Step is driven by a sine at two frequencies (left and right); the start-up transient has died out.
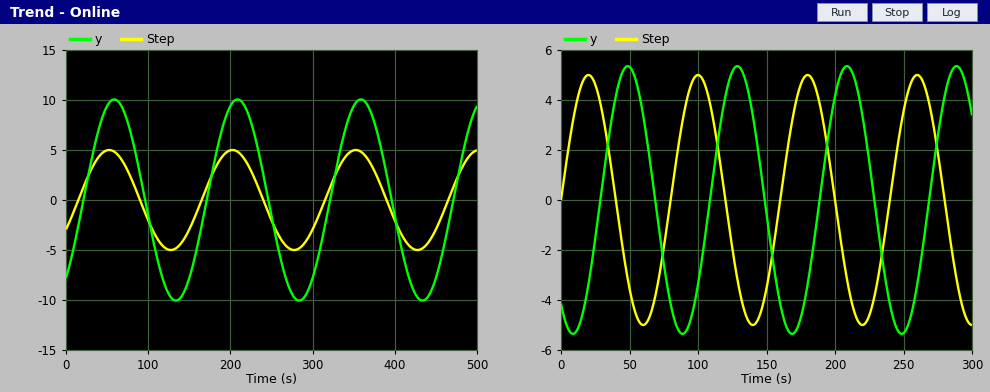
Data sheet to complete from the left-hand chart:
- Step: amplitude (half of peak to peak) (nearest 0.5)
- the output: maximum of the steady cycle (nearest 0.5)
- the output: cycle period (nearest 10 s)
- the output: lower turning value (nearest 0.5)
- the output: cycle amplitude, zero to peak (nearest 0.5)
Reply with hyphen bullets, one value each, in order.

- 5.0
- 10.0
- 150 s
- -10.0
- 10.0
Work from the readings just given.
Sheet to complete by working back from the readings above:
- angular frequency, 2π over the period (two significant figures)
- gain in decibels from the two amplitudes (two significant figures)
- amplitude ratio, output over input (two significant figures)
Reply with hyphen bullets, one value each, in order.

- 0.042 rad/s
- 6.0 dB
- 2.0
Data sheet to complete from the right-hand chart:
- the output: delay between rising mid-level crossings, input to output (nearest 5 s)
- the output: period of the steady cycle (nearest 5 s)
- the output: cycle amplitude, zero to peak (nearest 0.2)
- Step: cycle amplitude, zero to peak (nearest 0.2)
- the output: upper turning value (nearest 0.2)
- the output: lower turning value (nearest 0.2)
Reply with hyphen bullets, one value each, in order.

- 30 s
- 80 s
- 5.4
- 5.0
- 5.4
- -5.4
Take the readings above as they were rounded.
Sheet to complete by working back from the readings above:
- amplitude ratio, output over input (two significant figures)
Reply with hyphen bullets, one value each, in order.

- 1.1
